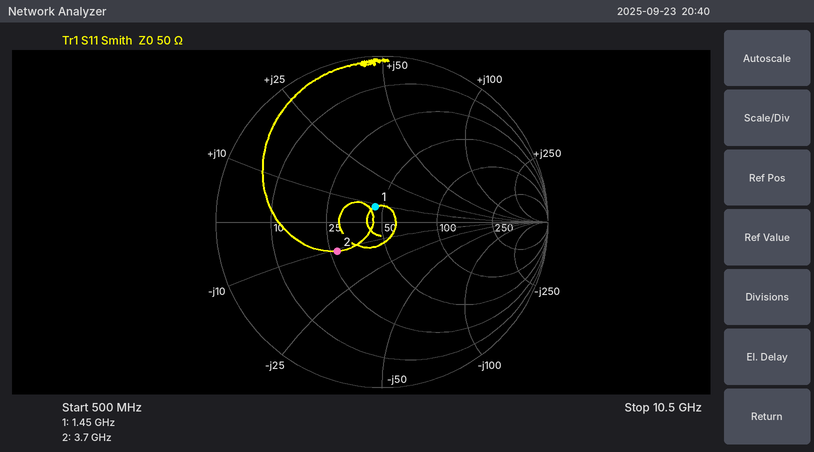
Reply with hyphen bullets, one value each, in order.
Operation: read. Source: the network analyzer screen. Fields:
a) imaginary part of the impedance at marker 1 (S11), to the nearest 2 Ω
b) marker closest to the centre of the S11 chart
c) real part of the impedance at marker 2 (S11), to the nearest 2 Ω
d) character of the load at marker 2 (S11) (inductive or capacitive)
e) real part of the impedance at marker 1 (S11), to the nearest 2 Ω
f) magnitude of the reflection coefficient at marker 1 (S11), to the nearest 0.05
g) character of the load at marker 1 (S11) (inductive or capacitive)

- +8 Ω
- marker 1
- 28 Ω
- capacitive
- 46 Ω
- 0.10
- inductive
